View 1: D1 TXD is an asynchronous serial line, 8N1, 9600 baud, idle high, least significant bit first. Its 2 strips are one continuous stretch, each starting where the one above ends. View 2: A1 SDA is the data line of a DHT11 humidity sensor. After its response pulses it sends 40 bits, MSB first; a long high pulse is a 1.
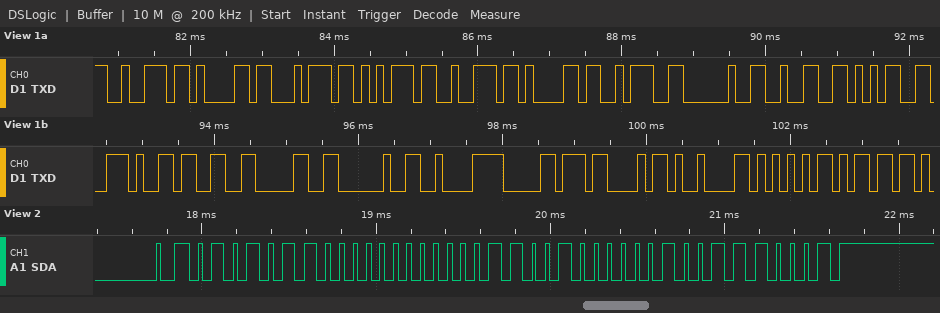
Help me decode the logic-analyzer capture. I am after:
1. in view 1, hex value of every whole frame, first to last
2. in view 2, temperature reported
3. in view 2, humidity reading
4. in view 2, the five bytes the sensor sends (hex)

72 61 74 75 72 61 3A 20 32 35 2E 33 30 20 C2 B0 43 09 55 6D
25.2 °C
86 %
56 00 19 02 71
